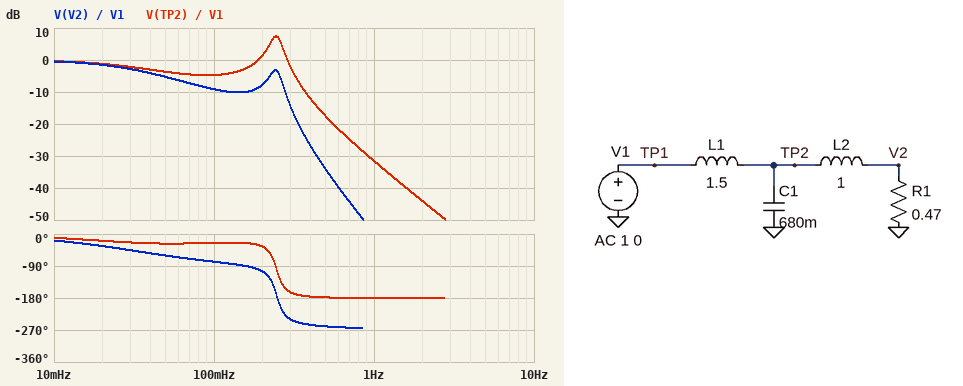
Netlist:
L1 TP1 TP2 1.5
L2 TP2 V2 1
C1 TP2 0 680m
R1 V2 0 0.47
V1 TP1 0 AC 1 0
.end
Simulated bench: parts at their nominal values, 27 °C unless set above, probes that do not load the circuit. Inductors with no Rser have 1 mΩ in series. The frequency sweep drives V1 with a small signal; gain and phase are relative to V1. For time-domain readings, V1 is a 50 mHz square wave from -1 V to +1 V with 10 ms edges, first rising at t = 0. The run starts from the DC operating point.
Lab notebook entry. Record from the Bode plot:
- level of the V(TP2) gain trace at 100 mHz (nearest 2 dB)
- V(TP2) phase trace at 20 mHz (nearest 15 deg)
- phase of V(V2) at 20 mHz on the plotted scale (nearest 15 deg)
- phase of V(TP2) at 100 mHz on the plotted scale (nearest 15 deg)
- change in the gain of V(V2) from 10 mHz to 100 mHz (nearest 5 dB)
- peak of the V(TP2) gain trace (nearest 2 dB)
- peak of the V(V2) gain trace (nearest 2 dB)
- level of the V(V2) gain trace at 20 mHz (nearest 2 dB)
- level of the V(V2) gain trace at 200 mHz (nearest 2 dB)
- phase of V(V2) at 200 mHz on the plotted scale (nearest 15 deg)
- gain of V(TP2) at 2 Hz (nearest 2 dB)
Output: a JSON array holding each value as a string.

["-4 dB", "-15 deg", "-30 deg", "-30 deg", "-10 dB", "8 dB", "0 dB", "-2 dB", "-8 dB", "-105 deg", "-44 dB"]
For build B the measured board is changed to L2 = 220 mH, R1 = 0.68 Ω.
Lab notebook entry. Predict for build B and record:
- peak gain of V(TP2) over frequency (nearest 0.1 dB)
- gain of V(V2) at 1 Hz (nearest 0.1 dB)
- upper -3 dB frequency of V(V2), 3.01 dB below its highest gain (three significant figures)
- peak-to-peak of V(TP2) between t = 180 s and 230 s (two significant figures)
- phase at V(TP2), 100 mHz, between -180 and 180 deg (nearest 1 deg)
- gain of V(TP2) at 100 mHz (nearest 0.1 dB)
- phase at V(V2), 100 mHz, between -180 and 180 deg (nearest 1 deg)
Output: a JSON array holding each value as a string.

["0 dB", "-37.7 dB", "77.8 mHz", "2.0 V", "-57 deg", "-4.0 dB", "-68 deg"]
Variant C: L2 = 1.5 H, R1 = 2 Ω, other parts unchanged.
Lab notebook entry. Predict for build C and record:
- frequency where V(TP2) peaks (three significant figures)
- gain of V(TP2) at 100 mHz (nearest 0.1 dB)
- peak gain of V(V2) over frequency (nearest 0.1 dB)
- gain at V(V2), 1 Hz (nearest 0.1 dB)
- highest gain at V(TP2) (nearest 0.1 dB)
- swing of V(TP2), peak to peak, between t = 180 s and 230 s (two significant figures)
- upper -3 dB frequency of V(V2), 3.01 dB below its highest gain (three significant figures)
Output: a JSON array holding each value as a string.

["188 mHz", "1.2 dB", "3.6 dB", "-45.3 dB", "6.1 dB", "3.3 V", "219 mHz"]
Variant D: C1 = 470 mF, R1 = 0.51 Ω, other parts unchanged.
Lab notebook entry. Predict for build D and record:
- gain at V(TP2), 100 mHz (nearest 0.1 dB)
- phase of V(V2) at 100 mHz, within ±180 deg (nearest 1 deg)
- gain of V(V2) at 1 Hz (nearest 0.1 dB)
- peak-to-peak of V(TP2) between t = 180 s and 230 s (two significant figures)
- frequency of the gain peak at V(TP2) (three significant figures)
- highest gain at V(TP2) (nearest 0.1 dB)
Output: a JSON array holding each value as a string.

["-5.0 dB", "-75 deg", "-49.9 dB", "2.0 V", "295 mHz", "8.3 dB"]
